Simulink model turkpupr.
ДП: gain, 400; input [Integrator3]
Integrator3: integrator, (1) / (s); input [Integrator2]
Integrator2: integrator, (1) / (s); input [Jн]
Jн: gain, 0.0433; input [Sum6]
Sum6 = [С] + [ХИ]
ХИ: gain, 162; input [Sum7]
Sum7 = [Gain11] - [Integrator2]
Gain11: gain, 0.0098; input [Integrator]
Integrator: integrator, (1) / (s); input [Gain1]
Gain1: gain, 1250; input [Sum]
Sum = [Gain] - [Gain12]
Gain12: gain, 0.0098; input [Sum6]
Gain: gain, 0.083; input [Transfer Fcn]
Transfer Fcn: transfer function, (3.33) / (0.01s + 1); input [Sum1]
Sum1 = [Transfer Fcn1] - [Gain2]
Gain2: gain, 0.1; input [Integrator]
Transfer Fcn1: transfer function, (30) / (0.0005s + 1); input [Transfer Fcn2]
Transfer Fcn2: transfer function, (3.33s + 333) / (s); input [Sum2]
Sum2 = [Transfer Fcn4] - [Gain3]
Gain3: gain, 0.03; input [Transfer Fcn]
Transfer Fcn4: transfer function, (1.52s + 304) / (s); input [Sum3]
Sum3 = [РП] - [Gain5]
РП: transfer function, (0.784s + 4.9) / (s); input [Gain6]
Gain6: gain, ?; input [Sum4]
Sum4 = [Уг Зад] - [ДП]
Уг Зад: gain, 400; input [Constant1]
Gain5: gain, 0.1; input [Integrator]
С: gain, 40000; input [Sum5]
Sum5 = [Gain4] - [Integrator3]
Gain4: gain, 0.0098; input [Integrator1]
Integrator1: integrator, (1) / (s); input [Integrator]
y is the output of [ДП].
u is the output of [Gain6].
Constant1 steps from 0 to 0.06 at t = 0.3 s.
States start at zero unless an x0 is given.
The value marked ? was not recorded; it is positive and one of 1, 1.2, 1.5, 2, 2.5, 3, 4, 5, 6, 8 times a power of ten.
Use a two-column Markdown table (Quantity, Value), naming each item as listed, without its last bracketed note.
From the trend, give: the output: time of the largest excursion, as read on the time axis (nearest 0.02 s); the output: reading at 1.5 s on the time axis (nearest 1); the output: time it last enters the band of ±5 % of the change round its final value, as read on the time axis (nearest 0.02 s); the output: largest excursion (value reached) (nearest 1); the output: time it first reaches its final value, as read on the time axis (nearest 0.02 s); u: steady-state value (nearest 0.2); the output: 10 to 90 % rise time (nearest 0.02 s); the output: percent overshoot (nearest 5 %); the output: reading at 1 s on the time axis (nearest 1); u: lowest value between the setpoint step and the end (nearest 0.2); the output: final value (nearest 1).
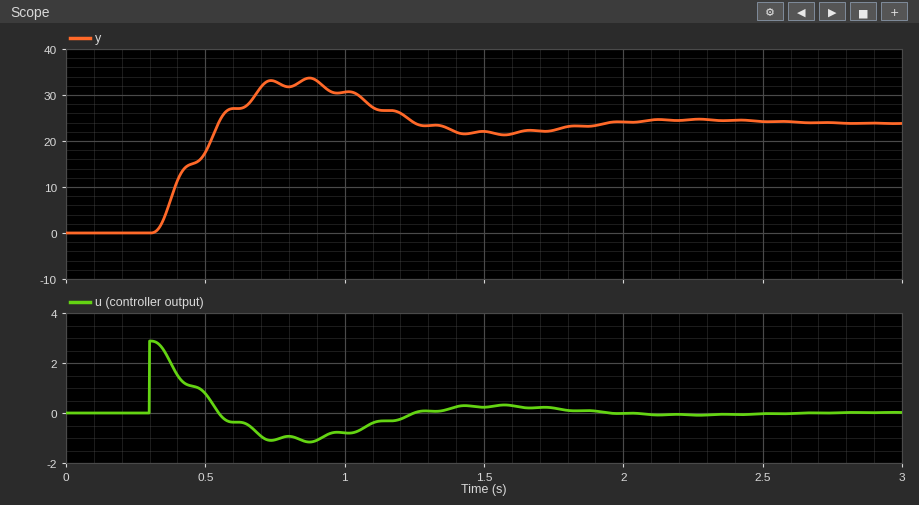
| Quantity | Value |
|---|---|
| the output: time of the largest excursion, as read on the time axis | 0.88 s |
| the output: reading at 1.5 s on the time axis | 22 |
| the output: time it last enters the band of ±5 % of the change round its final value, as read on the time axis | 1.78 s |
| the output: largest excursion (value reached) | 34 |
| the output: time it first reaches its final value, as read on the time axis | 0.54 s |
| u: steady-state value | 0.0 |
| the output: 10 to 90 % rise time | 0.18 s |
| the output: percent overshoot | 40 % |
| the output: reading at 1 s on the time axis | 31 |
| u: lowest value between the setpoint step and the end | -1.2 |
| the output: final value | 24 |
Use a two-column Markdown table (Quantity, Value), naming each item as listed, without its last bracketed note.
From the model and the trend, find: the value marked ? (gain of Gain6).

| Quantity | Value |
|---|---|
| the value marked ? | 0.12 |
